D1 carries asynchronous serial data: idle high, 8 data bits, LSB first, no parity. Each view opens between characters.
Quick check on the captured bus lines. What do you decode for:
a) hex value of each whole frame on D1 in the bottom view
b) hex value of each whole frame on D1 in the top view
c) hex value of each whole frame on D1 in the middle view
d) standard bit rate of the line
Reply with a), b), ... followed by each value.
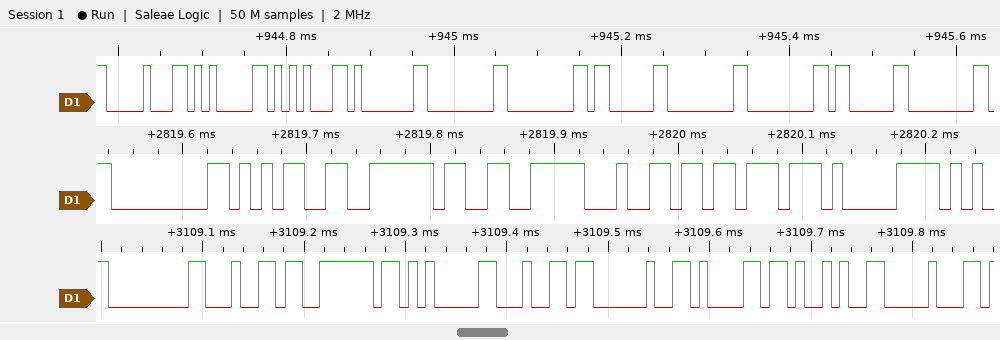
a) 00, 64, 7E, 05, 64, 20, 61, 29, 10
b) 10, 05, 15, 01, 00, 00, 03, 00, 00, 03, 00
c) 00, 35, 7E, E6, 64, BB, C1
d) 115200 baud
